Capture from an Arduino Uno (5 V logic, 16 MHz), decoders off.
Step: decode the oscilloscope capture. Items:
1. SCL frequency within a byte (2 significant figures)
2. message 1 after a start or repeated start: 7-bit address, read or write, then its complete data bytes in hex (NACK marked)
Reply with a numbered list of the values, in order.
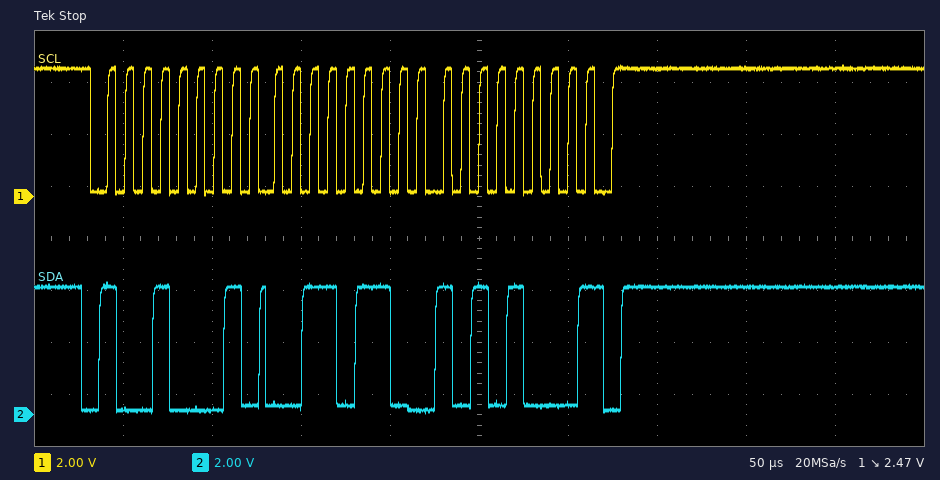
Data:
1. 100 kHz
2. 0x48 read: 36 A8 NACK
